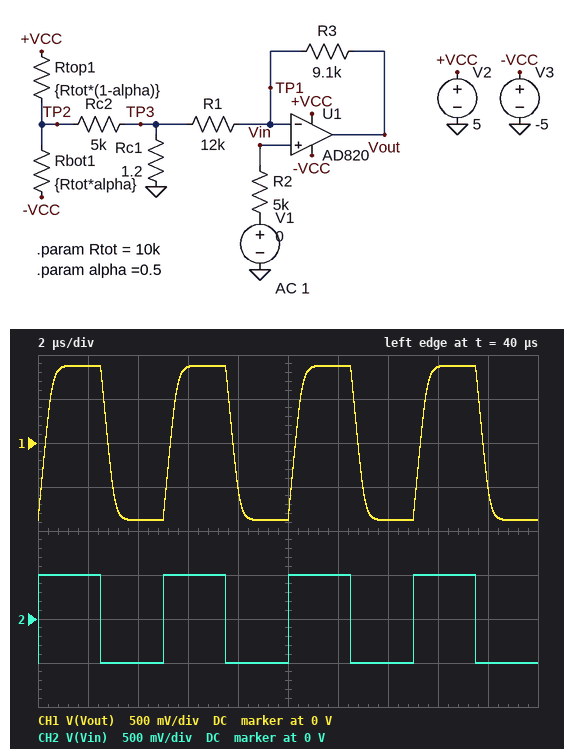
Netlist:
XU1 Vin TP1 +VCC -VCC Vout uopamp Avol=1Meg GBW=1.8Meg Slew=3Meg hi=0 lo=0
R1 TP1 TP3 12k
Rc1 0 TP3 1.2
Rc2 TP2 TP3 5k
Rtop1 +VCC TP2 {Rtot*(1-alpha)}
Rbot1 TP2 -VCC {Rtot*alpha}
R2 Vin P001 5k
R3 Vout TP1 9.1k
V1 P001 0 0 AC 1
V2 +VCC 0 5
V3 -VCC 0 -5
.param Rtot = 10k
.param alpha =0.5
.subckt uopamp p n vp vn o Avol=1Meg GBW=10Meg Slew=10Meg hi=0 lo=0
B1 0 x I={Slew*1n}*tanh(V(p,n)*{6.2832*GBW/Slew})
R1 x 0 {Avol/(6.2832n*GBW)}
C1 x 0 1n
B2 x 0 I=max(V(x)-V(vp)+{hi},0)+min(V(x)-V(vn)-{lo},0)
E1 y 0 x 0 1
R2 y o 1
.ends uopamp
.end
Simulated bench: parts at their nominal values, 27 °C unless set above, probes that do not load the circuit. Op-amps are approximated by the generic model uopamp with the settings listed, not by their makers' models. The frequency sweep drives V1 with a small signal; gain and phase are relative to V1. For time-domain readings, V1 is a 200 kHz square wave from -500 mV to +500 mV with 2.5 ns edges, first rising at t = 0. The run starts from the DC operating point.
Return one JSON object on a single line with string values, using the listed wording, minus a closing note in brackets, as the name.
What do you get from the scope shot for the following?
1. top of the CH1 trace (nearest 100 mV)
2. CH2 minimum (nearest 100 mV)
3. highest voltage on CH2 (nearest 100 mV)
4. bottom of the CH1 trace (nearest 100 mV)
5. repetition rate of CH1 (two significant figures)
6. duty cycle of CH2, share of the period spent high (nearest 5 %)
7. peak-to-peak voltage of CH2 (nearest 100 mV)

{"top of the CH1 trace": "900 mV", "CH2 minimum": "-500 mV", "highest voltage on CH2": "500 mV", "bottom of the CH1 trace": "-900 mV", "repetition rate of CH1": "200 kHz", "duty cycle of CH2, share of the period spent high": "50 %", "peak-to-peak voltage of CH2": "1.0 V"}
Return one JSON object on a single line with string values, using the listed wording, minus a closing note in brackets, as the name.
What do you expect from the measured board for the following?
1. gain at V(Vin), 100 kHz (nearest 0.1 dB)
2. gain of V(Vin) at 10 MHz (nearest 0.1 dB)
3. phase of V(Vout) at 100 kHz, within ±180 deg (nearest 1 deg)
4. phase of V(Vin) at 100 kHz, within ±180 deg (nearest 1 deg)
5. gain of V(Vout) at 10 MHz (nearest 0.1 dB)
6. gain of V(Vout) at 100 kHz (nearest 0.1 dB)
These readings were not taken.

{"gain at V(Vin), 100 kHz": "0 dB", "gain of V(Vin) at 10 MHz": "0 dB", "phase of V(Vout) at 100 kHz, within ±180 deg": "-6 deg", "phase of V(Vin) at 100 kHz, within ±180 deg": "0 deg", "gain of V(Vout) at 10 MHz": "-14.9 dB", "gain of V(Vout) at 100 kHz": "4.9 dB"}
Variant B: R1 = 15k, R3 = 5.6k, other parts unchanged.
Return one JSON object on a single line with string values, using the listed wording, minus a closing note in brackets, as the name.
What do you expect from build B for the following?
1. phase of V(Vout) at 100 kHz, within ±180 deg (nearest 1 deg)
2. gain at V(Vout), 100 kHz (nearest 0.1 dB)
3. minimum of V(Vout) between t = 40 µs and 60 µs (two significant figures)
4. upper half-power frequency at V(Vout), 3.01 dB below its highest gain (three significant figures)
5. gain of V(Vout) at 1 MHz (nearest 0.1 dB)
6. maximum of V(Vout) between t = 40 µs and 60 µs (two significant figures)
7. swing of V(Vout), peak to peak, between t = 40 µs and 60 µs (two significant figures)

{"phase of V(Vout) at 100 kHz, within ±180 deg": "-4 deg", "gain at V(Vout), 100 kHz": "2.7 dB", "minimum of V(Vout) between t = 40 µs and 60 µs": "-690 mV", "upper half-power frequency at V(Vout), 3.01 dB below its highest gain": "1.31 MHz", "gain of V(Vout) at 1 MHz": "0.8 dB", "maximum of V(Vout) between t = 40 µs and 60 µs": "690 mV", "swing of V(Vout), peak to peak, between t = 40 µs and 60 µs": "1.4 V"}
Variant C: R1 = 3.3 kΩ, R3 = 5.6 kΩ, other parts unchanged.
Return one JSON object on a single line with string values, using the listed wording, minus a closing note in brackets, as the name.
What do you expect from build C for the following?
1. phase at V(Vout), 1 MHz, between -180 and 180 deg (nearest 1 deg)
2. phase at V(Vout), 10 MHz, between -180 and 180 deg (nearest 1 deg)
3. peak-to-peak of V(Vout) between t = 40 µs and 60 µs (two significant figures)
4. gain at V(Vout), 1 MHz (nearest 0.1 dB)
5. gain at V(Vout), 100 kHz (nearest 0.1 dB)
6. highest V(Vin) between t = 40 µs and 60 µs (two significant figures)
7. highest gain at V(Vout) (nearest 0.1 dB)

{"phase at V(Vout), 1 MHz, between -180 and 180 deg": "-56 deg", "phase at V(Vout), 10 MHz, between -180 and 180 deg": "-86 deg", "peak-to-peak of V(Vout) between t = 40 µs and 60 µs": "2.7 V", "gain at V(Vout), 1 MHz": "3.5 dB", "gain at V(Vout), 100 kHz": "8.5 dB", "highest V(Vin) between t = 40 µs and 60 µs": "500 mV", "highest gain at V(Vout)": "8.6 dB"}
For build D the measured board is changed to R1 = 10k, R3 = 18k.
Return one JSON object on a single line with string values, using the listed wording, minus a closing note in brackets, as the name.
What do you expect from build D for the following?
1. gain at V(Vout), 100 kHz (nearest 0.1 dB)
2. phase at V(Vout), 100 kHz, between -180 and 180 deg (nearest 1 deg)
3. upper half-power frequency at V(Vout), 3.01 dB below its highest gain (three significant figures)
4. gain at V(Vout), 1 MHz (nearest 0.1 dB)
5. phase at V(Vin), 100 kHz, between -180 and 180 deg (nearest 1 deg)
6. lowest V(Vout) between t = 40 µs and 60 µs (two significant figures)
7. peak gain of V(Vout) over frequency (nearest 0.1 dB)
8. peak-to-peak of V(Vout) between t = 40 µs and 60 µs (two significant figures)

{"gain at V(Vout), 100 kHz": "8.8 dB", "phase at V(Vout), 100 kHz, between -180 and 180 deg": "-9 deg", "upper half-power frequency at V(Vout), 3.01 dB below its highest gain": "643 kHz", "gain at V(Vout), 1 MHz": "3.6 dB", "phase at V(Vin), 100 kHz, between -180 and 180 deg": "0 deg", "lowest V(Vout) between t = 40 µs and 60 µs": "-1.4 V", "peak gain of V(Vout) over frequency": "8.9 dB", "peak-to-peak of V(Vout) between t = 40 µs and 60 µs": "2.8 V"}
